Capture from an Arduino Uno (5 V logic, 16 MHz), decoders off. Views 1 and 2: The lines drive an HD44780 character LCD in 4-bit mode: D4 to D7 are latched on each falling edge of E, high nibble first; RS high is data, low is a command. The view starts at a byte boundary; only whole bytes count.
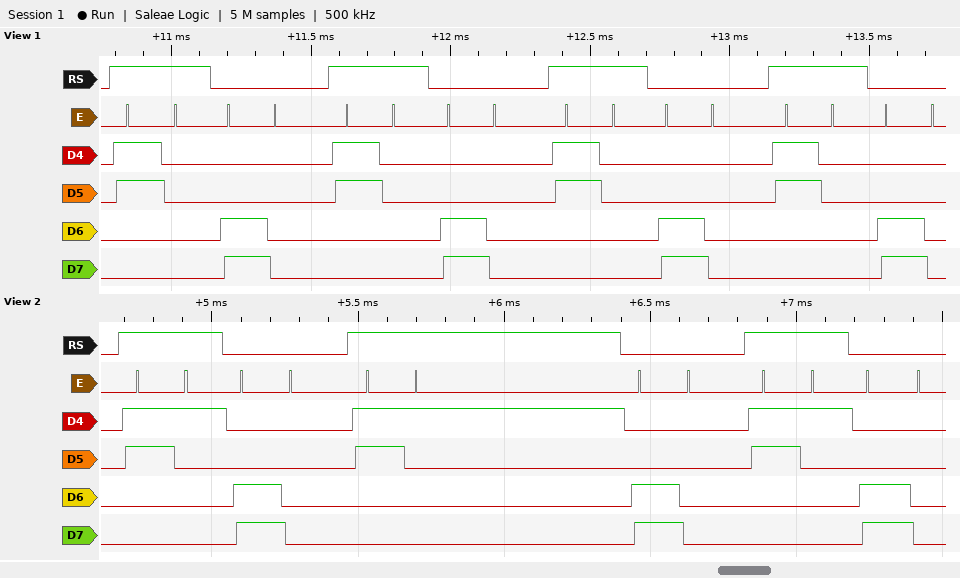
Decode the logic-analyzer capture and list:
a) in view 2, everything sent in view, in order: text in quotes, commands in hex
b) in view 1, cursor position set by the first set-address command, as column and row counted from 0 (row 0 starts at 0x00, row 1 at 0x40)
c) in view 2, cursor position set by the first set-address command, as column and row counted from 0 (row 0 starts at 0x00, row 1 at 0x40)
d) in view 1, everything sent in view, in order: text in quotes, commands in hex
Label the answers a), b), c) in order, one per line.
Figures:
a) "1" 0xC0 "1" 0xC0 "1" 0xC0
b) column 0, row 1
c) column 0, row 1
d) "0" 0xC0 "0" 0xC0 "0" 0xC0 "0" 0xC0
